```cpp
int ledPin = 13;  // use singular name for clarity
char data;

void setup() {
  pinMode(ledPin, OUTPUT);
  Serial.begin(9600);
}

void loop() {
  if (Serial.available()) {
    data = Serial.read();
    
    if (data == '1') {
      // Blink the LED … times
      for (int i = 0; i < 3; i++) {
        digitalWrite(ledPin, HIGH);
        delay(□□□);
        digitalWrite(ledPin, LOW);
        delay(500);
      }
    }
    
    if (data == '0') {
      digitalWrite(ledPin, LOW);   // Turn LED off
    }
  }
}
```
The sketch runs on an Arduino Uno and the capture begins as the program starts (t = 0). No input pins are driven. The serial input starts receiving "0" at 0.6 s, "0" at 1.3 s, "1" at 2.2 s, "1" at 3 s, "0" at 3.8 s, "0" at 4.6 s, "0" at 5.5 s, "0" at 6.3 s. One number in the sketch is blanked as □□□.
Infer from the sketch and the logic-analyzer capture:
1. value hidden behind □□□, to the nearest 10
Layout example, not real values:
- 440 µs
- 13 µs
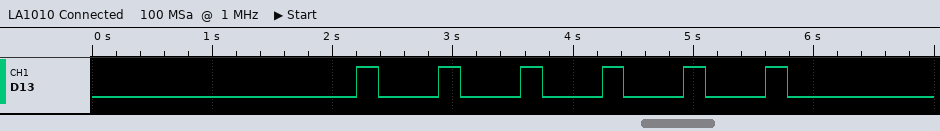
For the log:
- 180
